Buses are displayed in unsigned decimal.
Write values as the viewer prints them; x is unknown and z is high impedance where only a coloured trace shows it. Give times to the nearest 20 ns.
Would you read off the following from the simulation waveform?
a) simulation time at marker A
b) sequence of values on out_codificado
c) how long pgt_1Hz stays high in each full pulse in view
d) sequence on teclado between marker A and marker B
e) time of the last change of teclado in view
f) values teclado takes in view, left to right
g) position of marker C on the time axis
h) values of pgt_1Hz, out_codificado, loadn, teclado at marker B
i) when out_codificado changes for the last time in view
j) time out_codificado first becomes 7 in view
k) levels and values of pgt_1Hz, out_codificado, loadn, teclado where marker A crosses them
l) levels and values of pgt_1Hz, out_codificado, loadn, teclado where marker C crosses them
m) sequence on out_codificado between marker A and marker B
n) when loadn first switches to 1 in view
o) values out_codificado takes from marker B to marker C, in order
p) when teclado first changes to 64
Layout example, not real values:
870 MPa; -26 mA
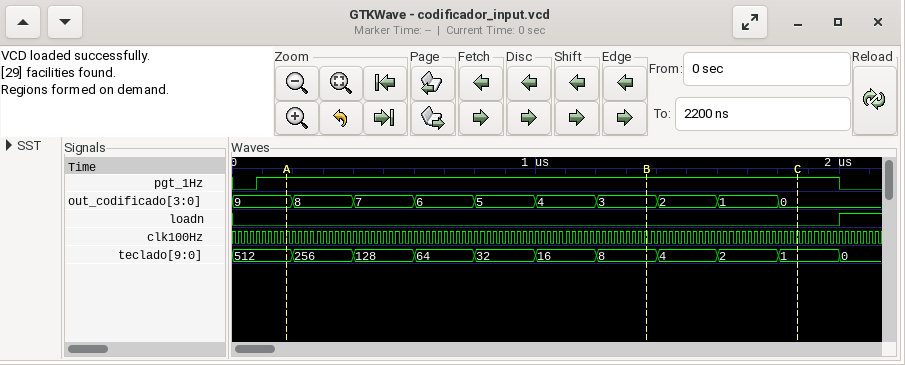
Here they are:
180 ns; 9, 8, 7, 6, 5, 4, 3, 2, 1, 0; 1920 ns; 512, 256, 128, 64, 32, 16, 8; 2000 ns; 512, 256, 128, 64, 32, 16, 8, 4, 2, 1, 0; 1860 ns; pgt_1Hz=1, out_codificado=3, loadn=0, teclado=8; 1800 ns; 400 ns; pgt_1Hz=1, out_codificado=9, loadn=0, teclado=512; pgt_1Hz=1, out_codificado=0, loadn=0, teclado=1; 9, 8, 7, 6, 5, 4, 3; 2000 ns; 3, 2, 1, 0; 600 ns
